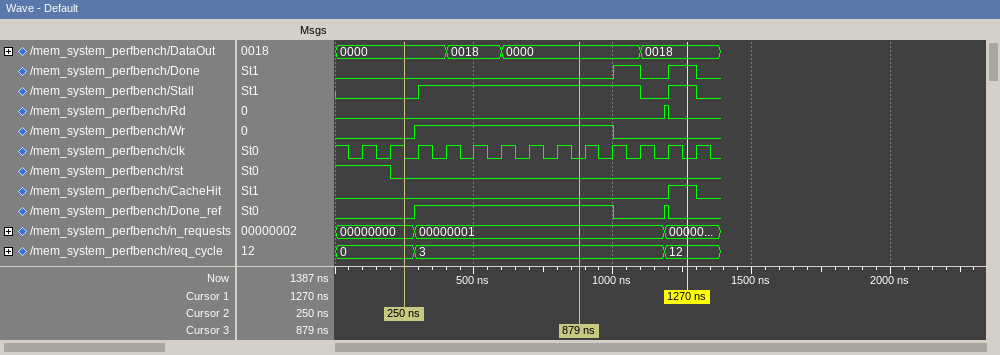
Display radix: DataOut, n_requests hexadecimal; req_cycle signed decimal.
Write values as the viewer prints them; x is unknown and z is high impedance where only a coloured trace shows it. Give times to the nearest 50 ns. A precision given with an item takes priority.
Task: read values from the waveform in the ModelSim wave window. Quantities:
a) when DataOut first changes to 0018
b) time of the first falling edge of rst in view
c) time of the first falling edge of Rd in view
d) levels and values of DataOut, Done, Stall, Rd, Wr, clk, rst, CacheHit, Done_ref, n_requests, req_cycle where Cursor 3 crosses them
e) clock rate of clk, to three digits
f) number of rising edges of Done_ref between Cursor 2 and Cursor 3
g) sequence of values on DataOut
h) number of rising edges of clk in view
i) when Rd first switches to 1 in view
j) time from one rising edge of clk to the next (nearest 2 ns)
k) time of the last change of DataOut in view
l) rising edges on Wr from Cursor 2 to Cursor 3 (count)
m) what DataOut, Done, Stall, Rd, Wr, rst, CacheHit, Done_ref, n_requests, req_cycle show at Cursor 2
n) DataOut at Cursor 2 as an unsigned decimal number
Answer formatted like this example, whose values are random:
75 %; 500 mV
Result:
400 ns; 200 ns; 1200 ns; DataOut=0000, Done=0, Stall=1, Rd=0, Wr=1, clk=0, rst=0, CacheHit=0, Done_ref=1, n_requests=00000001, req_cycle=3; 10.0 MHz; 1; 0000, 0018, 0000, 0018; 13; 1200 ns; 100 ns; 1100 ns; 1; DataOut=0000, Done=0, Stall=0, Rd=0, Wr=0, rst=0, CacheHit=0, Done_ref=0, n_requests=00000000, req_cycle=0; 0
